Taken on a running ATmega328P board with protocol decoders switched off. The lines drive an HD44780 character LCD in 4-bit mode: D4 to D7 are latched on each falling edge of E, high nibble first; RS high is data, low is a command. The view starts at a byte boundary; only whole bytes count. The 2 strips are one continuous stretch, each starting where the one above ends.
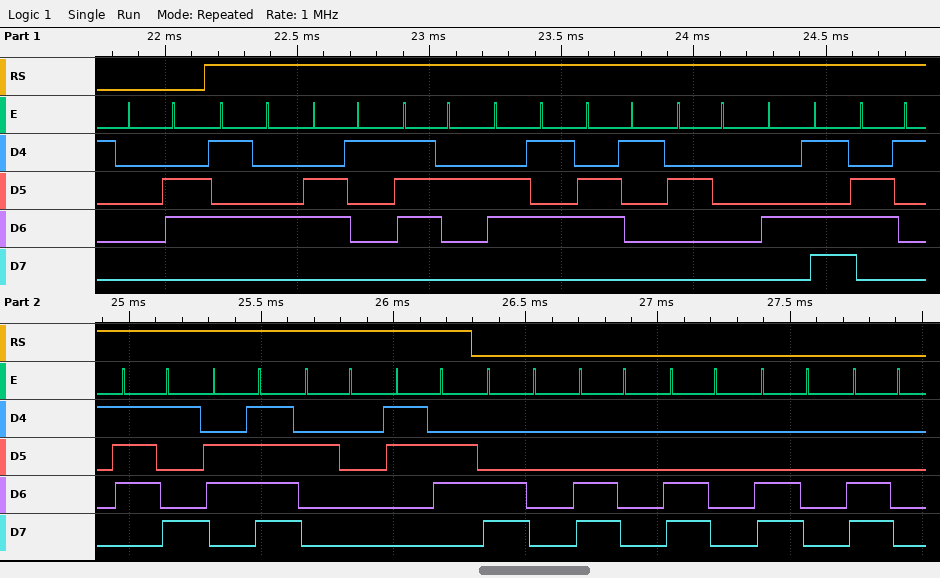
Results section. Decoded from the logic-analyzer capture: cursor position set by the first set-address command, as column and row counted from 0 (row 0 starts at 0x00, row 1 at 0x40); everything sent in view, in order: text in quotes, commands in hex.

column 0, row 1
0x06 "Tarea Mayo 6" 0xC0 0xC0 0xC0 0xC0 0xC0
